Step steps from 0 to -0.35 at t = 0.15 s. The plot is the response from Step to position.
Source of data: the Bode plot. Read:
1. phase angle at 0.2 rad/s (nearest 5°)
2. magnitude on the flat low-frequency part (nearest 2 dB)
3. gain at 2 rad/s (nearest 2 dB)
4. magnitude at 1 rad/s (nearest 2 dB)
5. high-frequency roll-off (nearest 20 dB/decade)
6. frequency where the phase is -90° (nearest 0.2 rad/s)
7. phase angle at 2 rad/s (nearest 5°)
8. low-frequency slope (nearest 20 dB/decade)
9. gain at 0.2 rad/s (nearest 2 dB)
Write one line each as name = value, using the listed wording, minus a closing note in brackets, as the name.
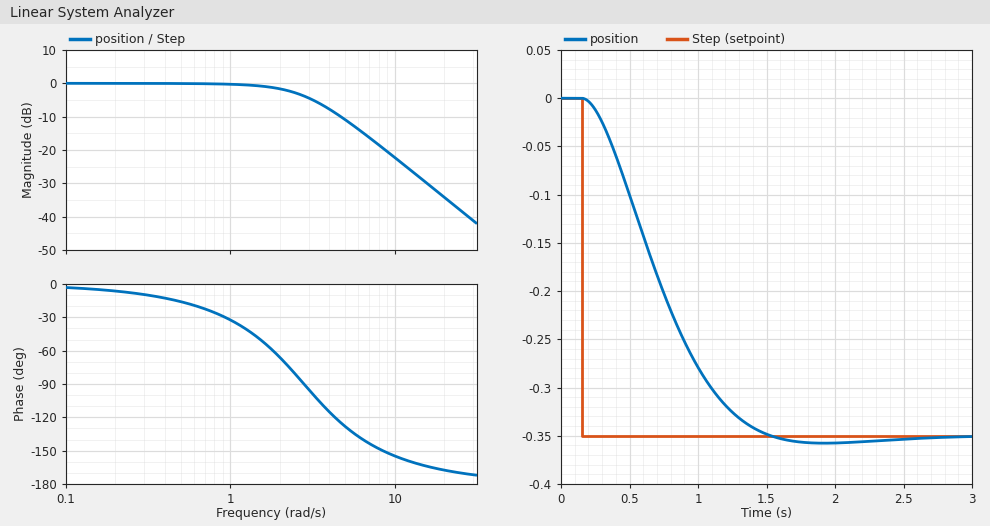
phase angle at 0.2 rad/s = -5°
magnitude on the flat low-frequency part = 0 dB
gain at 2 rad/s = -2 dB
magnitude at 1 rad/s = 0 dB
high-frequency roll-off = -40 dB/decade
frequency where the phase is -90° = 2.8 rad/s
phase angle at 2 rad/s = -65°
low-frequency slope = 0 dB/decade
gain at 0.2 rad/s = 0 dB
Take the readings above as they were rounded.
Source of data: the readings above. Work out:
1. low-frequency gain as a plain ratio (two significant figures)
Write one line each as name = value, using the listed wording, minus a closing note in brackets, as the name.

low-frequency gain as a plain ratio = 1.0
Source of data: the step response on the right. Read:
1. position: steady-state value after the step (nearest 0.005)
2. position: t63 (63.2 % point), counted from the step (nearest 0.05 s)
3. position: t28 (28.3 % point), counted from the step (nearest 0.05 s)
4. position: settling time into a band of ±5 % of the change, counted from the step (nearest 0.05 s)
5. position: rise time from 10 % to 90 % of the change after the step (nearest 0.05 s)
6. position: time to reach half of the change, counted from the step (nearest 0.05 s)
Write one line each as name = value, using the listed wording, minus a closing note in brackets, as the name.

position: steady-state value after the step = -0.350
position: t63 (63.2 % point), counted from the step = 0.65 s
position: t28 (28.3 % point), counted from the step = 0.35 s
position: settling time into a band of ±5 % of the change, counted from the step = 1.15 s
position: rise time from 10 % to 90 % of the change after the step = 0.85 s
position: time to reach half of the change, counted from the step = 0.55 s
